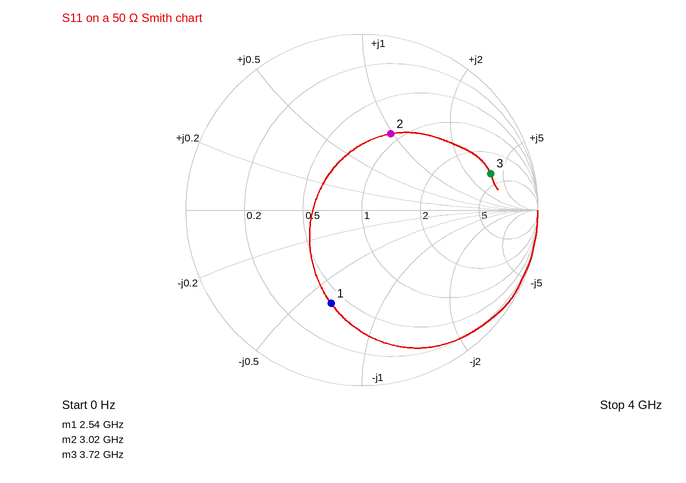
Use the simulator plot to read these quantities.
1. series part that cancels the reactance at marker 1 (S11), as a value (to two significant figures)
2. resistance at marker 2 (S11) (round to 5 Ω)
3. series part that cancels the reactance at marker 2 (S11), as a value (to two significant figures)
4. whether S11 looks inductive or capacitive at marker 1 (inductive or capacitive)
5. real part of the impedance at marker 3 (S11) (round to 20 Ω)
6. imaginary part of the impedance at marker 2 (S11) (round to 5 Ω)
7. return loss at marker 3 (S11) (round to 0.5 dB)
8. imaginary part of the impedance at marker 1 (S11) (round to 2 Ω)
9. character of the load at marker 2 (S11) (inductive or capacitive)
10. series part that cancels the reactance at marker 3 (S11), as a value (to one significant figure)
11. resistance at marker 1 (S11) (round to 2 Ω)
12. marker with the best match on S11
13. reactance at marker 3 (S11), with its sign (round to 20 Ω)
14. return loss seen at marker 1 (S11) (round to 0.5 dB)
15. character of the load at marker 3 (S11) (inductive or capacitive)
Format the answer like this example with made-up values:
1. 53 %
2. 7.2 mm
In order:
1. 2.0 nH
2. 45 Ω
3. 1.1 pF
4. capacitive
5. 180 Ω
6. +50 Ω
7. 2.5 dB
8. -32 Ω
9. inductive
10. 200 fF
11. 20 Ω
12. marker 2
13. +180 Ω
14. 5.0 dB
15. inductive
